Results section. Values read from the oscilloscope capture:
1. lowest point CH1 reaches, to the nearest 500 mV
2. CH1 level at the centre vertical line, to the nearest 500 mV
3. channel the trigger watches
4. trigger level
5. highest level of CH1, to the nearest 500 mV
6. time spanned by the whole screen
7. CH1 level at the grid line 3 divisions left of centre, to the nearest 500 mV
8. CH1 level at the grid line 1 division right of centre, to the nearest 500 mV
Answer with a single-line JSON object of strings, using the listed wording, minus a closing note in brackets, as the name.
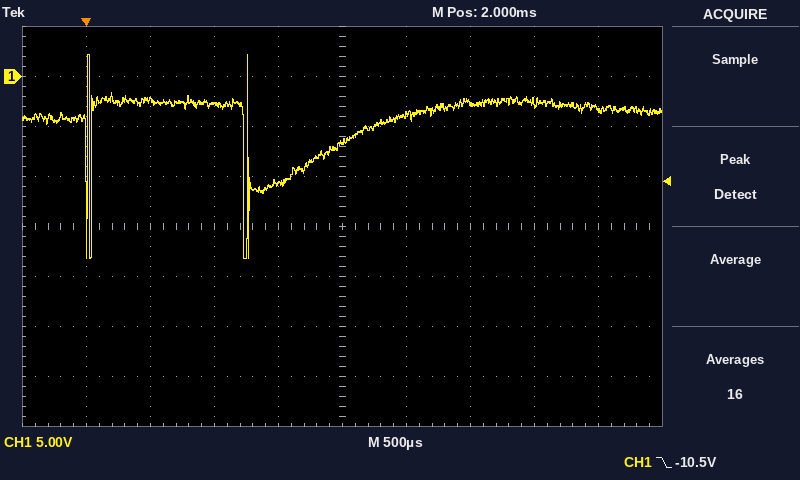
{"lowest point CH1 reaches, to the nearest 500 mV": "-18.0 V", "CH1 level at the centre vertical line, to the nearest 500 mV": "-6.5 V", "channel the trigger watches": "CH1", "trigger level": "-10.5 V", "highest level of CH1, to the nearest 500 mV": "2.0 V", "time spanned by the whole screen": "5 ms", "CH1 level at the grid line 3 divisions left of centre, to the nearest 500 mV": "-2.5 V", "CH1 level at the grid line 1 division right of centre, to the nearest 500 mV": "-4.0 V"}
